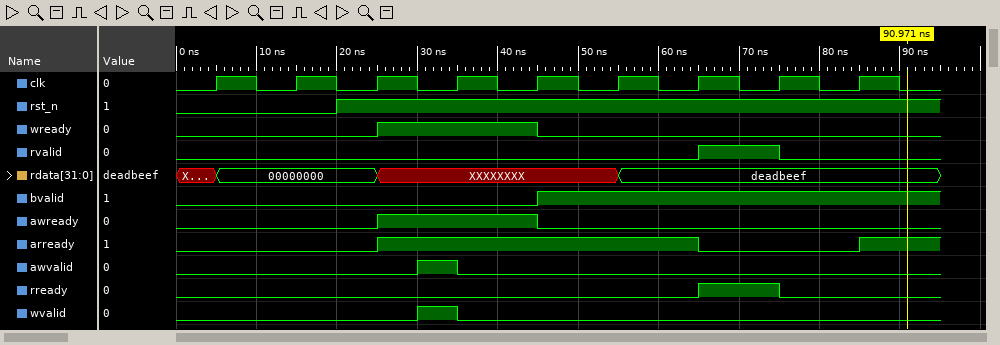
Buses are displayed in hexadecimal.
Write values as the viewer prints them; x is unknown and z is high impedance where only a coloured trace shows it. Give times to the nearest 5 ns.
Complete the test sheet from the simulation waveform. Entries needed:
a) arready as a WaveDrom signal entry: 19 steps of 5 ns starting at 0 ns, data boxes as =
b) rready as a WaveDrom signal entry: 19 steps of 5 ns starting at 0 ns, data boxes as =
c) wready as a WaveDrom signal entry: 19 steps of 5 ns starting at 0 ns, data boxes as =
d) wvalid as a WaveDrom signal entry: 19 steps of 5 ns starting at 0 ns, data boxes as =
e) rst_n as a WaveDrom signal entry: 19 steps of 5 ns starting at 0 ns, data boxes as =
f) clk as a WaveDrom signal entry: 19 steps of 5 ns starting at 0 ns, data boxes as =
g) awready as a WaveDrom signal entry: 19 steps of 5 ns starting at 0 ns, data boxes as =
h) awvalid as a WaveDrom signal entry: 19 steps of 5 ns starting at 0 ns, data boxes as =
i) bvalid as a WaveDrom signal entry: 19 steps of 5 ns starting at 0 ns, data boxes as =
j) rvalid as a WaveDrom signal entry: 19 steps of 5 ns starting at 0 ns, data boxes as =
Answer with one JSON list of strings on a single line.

["{name: 'arready', wave: '0....1.......0...1.'}", "{name: 'rready', wave: '0............1.0...'}", "{name: 'wready', wave: '0....1...0.........'}", "{name: 'wvalid', wave: '0.....10...........'}", "{name: 'rst_n', wave: '0...1..............'}", "{name: 'clk', wave: '0101010101010101010'}", "{name: 'awready', wave: '0....1...0.........'}", "{name: 'awvalid', wave: '0.....10...........'}", "{name: 'bvalid', wave: '0........1.........'}", "{name: 'rvalid', wave: '0............1.0...'}"]
